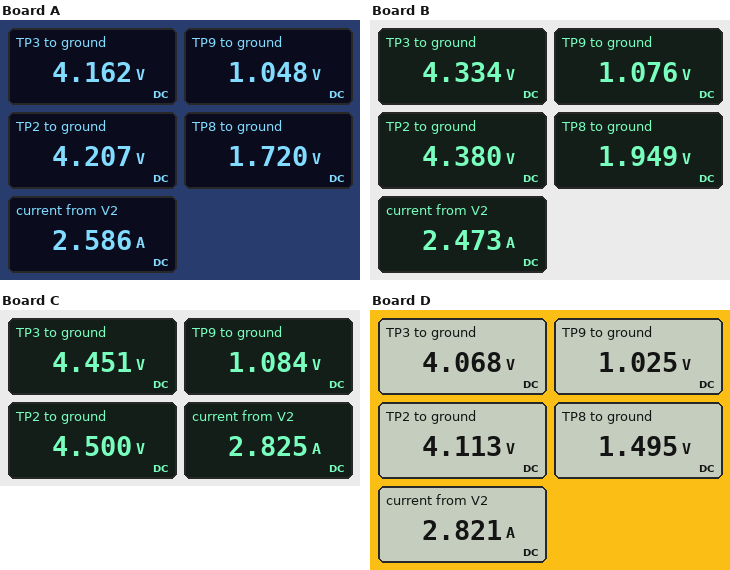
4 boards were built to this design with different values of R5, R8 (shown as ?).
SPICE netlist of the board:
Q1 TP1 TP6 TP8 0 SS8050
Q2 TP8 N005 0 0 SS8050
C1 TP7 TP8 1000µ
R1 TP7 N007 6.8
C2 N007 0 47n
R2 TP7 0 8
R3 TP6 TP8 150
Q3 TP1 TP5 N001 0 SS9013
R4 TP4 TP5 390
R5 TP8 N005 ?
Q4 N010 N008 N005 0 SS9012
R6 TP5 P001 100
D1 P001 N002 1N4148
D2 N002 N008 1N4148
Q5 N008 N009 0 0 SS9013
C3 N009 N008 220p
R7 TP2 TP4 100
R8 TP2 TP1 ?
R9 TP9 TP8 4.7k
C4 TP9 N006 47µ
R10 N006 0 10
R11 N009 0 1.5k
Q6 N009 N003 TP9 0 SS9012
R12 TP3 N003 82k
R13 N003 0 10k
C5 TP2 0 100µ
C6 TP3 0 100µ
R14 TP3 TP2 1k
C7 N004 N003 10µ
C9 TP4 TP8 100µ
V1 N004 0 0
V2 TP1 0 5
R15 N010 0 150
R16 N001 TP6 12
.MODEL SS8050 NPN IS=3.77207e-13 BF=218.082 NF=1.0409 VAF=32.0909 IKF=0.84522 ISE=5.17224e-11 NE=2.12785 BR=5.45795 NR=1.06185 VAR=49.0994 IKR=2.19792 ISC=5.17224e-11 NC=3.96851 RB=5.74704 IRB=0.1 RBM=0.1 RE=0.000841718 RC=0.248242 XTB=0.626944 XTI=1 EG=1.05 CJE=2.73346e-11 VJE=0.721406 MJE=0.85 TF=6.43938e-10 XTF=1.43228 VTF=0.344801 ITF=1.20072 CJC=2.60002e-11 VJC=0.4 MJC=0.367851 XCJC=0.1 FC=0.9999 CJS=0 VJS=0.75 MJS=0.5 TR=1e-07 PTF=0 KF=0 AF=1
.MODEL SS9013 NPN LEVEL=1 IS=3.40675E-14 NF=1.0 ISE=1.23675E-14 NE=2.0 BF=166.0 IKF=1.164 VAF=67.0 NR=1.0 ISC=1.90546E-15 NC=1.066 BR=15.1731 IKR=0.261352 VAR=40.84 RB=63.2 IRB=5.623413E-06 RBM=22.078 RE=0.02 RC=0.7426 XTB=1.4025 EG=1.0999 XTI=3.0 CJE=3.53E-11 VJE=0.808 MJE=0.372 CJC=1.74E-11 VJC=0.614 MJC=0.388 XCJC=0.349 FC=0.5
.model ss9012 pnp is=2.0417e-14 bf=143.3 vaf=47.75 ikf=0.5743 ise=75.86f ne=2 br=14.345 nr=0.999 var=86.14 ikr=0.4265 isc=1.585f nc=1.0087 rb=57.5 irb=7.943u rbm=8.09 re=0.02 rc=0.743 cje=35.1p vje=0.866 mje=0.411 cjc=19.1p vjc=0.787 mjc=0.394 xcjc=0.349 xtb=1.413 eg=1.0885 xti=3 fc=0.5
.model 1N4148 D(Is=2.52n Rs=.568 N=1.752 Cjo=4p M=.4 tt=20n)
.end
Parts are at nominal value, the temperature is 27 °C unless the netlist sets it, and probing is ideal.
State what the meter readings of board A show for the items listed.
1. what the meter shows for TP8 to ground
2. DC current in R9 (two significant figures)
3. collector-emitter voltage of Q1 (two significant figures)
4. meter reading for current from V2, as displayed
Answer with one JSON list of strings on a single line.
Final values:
["1.720 V", "140 µA", "3.3 V", "2.586 A"]
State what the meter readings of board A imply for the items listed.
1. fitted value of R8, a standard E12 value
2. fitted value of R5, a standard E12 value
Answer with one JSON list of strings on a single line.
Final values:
["2.2 kΩ", "15 Ω"]
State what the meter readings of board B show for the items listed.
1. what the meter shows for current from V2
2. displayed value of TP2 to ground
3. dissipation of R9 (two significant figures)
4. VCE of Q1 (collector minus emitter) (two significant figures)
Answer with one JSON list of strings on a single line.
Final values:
["2.473 A", "4.380 V", "160 µW", "3.1 V"]
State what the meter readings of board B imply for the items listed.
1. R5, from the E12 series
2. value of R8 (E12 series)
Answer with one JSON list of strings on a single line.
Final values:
["22 Ω", "1.8 kΩ"]
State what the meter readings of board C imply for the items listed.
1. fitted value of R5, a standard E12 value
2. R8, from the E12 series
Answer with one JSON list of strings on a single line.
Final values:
["15 Ω", "1.2 kΩ"]
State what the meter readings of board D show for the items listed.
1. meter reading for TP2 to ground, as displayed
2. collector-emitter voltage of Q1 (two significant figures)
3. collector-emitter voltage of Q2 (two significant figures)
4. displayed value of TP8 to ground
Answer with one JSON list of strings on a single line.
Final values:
["4.113 V", "3.5 V", "1.5 V", "1.495 V"]
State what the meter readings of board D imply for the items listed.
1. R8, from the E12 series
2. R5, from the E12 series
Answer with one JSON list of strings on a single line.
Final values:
["2.2 kΩ", "8.2 Ω"]
